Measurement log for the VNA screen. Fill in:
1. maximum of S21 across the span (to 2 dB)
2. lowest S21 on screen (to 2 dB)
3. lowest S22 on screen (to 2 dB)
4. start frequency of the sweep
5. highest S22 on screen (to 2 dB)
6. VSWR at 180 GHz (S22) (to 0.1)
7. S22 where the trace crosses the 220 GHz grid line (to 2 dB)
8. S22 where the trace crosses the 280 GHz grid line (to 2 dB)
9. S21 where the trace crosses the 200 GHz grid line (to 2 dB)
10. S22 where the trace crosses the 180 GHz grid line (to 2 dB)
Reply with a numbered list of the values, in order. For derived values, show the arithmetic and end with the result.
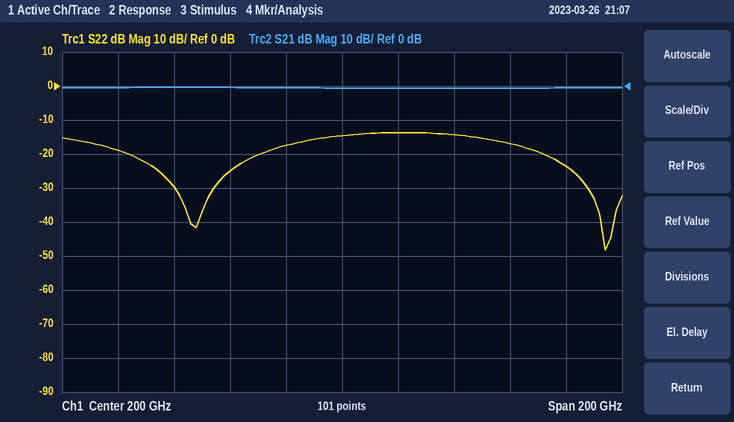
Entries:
1. 0 dB
2. 0 dB
3. -48 dB
4. 100 GHz
5. -14 dB
6. |Γ| = 10^(-18/20) = 0.1259; VSWR = (1 + 0.1259)/(1 − 0.1259) ≈ 1.3
7. -14 dB
8. -24 dB
9. 0 dB
10. -18 dB
